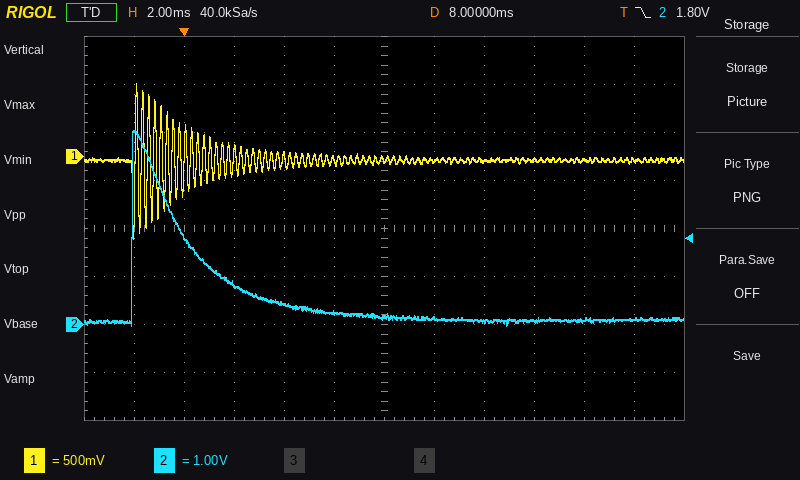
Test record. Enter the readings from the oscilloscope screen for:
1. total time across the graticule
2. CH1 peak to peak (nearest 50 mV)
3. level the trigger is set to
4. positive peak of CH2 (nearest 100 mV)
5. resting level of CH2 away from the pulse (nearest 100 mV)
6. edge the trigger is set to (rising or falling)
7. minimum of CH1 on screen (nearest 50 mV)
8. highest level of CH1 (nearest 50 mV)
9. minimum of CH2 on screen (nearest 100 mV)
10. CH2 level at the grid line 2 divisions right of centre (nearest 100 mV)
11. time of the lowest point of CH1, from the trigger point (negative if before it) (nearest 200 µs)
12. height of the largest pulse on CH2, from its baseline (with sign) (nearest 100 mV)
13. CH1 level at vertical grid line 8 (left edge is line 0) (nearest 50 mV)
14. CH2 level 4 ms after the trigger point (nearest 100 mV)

24 ms
1.60 V
1.80 V
4.0 V
100 mV
falling
-850 mV
750 mV
0.0 V
100 mV
-2.0 ms
+3.9 V
-50 mV
400 mV
